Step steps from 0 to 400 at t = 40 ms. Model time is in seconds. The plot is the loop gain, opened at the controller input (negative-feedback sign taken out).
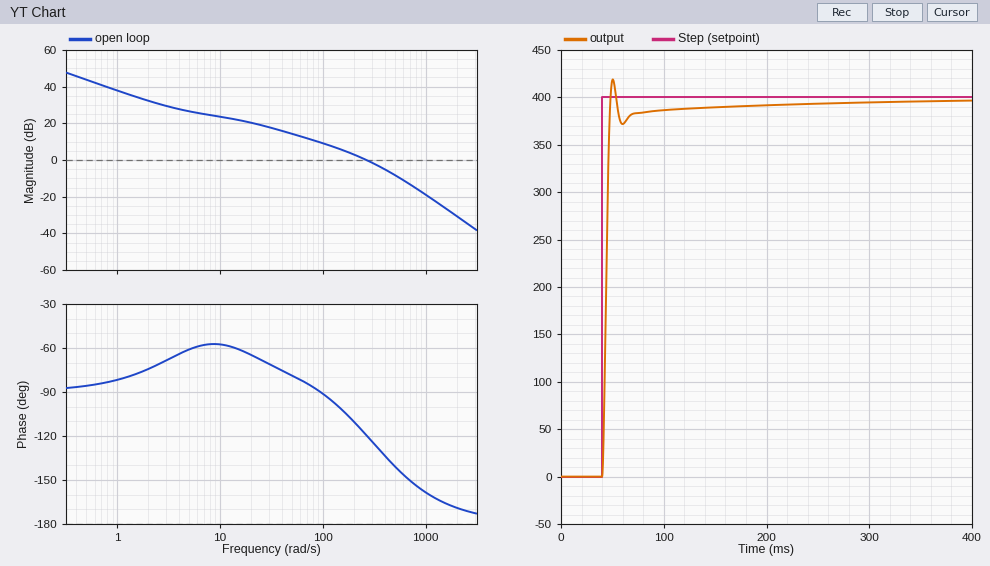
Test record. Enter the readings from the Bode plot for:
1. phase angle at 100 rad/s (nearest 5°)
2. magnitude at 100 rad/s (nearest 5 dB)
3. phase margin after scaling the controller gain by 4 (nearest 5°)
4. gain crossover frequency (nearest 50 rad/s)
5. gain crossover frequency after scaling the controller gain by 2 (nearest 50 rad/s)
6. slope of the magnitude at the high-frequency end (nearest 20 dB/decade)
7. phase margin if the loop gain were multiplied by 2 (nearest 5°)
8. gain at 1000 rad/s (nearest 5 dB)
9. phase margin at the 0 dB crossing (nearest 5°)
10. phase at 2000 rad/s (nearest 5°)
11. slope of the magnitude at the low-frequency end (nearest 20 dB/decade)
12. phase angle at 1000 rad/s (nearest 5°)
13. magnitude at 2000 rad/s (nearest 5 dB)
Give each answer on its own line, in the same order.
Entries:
-90°
10 dB
30°
250 rad/s
450 rad/s
-40 dB/decade
45°
-20 dB
60°
-170°
-20 dB/decade
-160°
-30 dB
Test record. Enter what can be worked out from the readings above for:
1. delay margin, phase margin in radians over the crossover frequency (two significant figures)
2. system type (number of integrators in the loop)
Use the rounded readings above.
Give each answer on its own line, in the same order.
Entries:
0.0042 s
1
